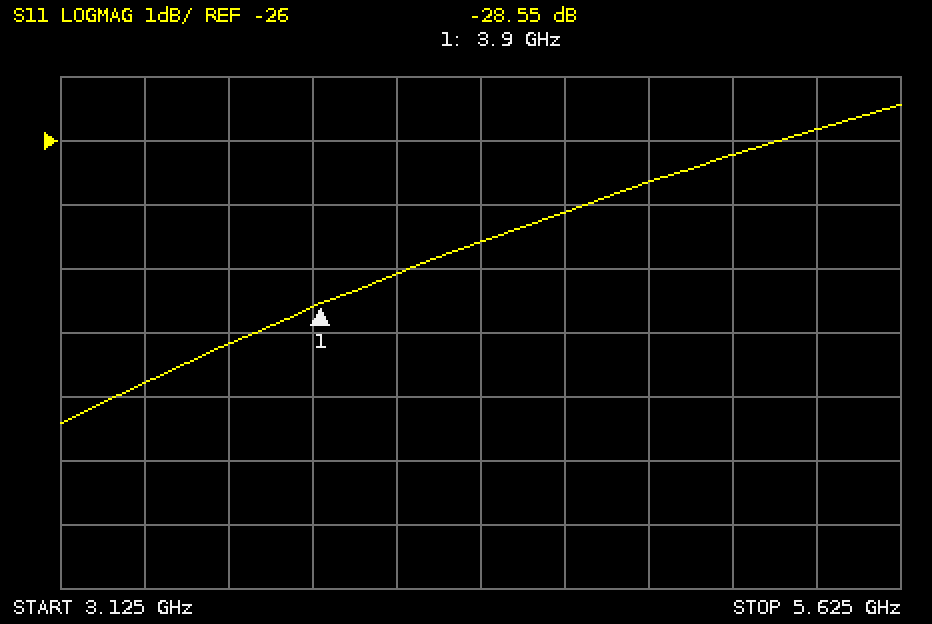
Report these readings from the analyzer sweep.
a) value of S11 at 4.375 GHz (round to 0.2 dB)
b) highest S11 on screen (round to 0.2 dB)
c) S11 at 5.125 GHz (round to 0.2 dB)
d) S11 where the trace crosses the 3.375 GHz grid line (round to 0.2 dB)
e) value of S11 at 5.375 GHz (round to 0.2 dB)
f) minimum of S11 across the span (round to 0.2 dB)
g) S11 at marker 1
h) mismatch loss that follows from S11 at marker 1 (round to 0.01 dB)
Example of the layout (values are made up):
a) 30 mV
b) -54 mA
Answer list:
a) -27.6 dB
b) -25.4 dB
c) -26.2 dB
d) -29.8 dB
e) -25.8 dB
f) -30.4 dB
g) -28.55 dB
h) 0.01 dB
